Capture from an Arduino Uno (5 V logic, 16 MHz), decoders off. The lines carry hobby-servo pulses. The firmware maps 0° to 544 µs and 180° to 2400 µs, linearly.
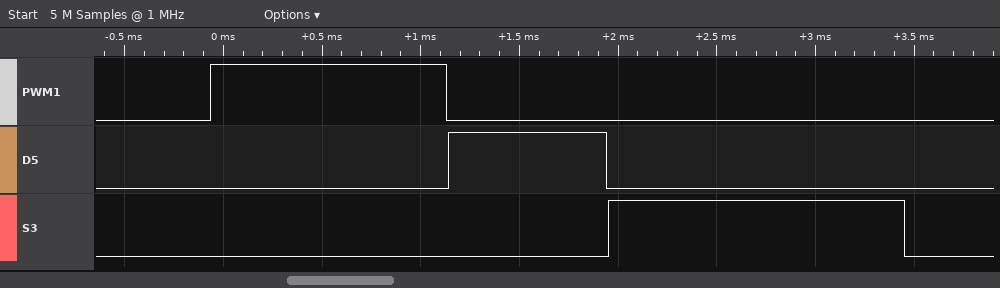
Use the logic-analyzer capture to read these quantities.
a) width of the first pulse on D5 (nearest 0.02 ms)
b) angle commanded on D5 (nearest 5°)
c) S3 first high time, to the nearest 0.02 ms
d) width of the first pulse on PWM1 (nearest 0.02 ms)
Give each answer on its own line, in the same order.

0.80 ms
25°
1.50 ms
1.20 ms
